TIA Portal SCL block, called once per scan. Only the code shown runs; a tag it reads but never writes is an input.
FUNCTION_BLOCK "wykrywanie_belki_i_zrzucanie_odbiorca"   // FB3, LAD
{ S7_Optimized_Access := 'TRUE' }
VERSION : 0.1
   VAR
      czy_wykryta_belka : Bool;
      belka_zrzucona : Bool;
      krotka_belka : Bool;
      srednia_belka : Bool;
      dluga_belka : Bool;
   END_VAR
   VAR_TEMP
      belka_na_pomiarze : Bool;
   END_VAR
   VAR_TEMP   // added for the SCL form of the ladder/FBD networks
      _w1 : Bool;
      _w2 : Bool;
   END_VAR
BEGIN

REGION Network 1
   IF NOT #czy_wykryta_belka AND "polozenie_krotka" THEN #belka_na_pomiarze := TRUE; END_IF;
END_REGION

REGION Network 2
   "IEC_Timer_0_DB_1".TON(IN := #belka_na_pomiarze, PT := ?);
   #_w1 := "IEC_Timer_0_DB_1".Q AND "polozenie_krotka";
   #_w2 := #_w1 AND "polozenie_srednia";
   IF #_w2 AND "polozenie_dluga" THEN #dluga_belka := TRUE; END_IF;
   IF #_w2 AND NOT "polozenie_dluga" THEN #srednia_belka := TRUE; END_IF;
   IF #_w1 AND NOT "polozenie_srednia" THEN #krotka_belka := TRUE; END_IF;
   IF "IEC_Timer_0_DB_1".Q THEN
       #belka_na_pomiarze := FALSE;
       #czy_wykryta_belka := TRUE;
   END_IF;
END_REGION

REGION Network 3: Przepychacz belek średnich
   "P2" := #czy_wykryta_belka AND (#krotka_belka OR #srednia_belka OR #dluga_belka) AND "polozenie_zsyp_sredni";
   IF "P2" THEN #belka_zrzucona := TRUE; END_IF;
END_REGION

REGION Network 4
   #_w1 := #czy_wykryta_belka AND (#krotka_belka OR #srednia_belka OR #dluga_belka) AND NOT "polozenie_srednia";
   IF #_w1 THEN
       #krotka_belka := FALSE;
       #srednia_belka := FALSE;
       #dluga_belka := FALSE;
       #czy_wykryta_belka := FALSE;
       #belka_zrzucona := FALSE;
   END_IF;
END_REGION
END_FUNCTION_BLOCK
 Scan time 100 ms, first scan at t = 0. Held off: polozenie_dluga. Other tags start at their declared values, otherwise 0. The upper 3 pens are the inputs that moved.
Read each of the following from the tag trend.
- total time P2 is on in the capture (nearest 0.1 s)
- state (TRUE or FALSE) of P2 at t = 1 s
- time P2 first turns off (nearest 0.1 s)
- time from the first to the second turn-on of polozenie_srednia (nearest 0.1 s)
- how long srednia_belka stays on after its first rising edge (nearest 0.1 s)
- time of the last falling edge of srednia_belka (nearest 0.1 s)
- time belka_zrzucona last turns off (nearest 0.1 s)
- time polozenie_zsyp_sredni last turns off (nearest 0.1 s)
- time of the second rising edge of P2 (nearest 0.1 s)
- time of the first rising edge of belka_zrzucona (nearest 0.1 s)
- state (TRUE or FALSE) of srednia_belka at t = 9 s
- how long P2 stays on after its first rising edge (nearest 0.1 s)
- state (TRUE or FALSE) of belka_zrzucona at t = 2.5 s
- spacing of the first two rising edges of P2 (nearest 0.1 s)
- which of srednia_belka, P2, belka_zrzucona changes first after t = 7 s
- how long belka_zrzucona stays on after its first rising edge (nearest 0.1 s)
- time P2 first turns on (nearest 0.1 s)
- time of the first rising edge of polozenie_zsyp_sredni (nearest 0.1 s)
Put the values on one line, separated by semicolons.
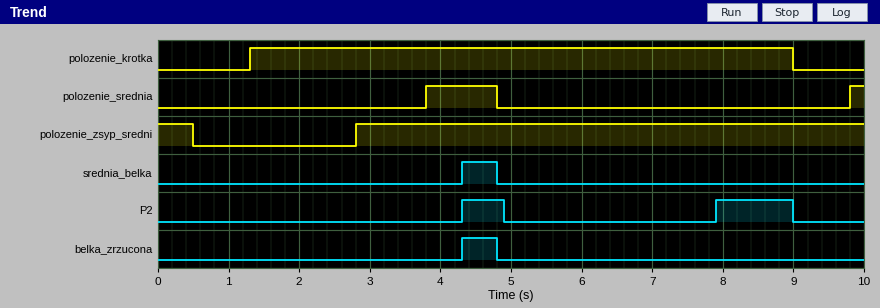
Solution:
1.7 s; FALSE; 4.9 s; 6.0 s; 0.5 s; 4.8 s; 4.8 s; 0.5 s; 7.9 s; 4.3 s; FALSE; 0.6 s; FALSE; 3.6 s; P2; 0.5 s; 4.3 s; 2.8 s
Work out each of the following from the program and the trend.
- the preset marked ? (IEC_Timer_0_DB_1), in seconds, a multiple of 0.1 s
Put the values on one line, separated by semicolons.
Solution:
3.0 s
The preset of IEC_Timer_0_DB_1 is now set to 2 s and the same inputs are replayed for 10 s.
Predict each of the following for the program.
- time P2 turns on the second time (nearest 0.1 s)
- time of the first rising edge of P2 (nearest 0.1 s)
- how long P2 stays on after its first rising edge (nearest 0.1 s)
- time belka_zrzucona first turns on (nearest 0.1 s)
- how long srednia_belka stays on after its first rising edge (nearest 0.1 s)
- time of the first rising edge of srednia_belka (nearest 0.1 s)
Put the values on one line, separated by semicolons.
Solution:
6.9 s; 3.3 s; 1.6 s; 3.8 s; 1.0 s; 3.8 s
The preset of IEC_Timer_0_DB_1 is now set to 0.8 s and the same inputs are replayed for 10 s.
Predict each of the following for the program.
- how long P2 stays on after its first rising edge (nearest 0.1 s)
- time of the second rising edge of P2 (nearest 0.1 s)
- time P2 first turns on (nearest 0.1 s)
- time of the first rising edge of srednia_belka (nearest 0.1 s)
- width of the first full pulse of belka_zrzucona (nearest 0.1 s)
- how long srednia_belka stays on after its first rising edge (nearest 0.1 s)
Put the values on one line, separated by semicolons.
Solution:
2.1 s; 5.7 s; 2.8 s; 3.8 s; 1.0 s; 1.0 s
